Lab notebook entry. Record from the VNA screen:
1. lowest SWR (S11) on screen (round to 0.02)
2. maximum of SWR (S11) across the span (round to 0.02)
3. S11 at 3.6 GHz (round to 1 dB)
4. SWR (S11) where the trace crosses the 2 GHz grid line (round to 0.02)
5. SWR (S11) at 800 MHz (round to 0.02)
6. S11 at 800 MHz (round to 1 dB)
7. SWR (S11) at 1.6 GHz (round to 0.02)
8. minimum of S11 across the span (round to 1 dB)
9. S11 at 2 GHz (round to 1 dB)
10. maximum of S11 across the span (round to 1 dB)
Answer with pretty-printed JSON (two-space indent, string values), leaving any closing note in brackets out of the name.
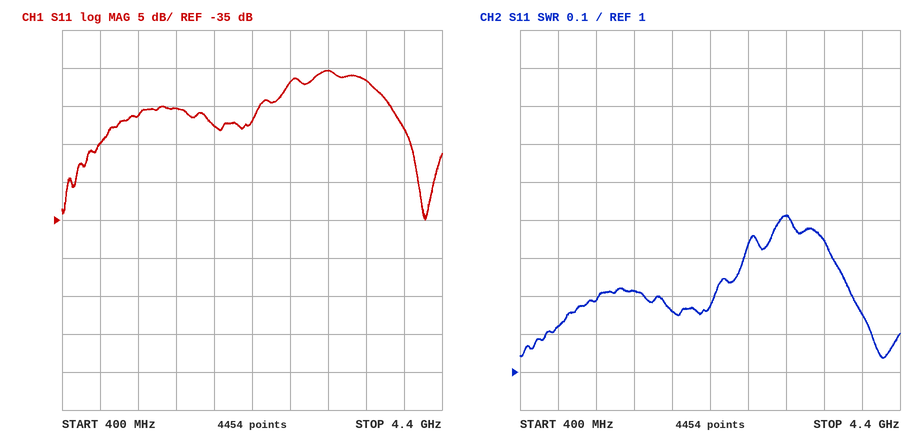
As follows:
{
  "lowest SWR (S11) on screen": "1.04",
  "maximum of SWR (S11) across the span": "1.42",
  "S11 at 3.6 GHz": "-17 dB",
  "SWR (S11) where the trace crosses the 2 GHz grid line": "1.16",
  "SWR (S11) at 800 MHz": "1.12",
  "S11 at 800 MHz": "-25 dB",
  "SWR (S11) at 1.6 GHz": "1.22",
  "minimum of S11 across the span": "-35 dB",
  "S11 at 2 GHz": "-23 dB",
  "maximum of S11 across the span": "-15 dB"
}
